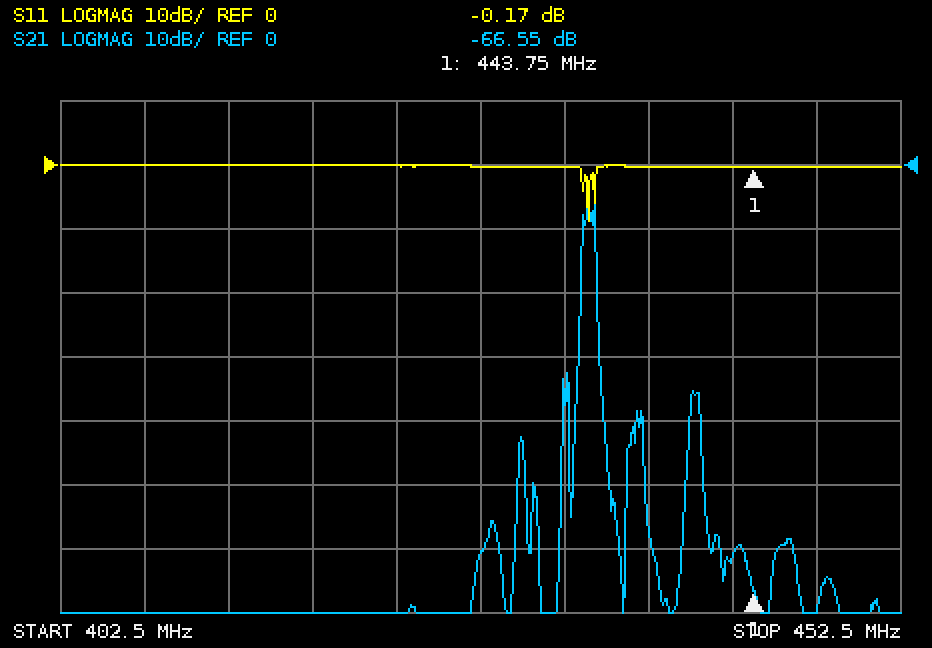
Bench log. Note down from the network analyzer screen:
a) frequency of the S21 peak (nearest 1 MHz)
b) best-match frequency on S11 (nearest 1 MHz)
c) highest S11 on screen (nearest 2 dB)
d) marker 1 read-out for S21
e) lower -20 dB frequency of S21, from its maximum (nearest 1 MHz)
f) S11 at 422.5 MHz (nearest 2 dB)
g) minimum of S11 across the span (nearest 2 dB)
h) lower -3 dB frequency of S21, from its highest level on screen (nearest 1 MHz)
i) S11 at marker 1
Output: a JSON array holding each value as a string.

["434 MHz", "434 MHz", "0 dB", "-66.55 dB", "433 MHz", "0 dB", "-8 dB", "434 MHz", "-0.17 dB"]
